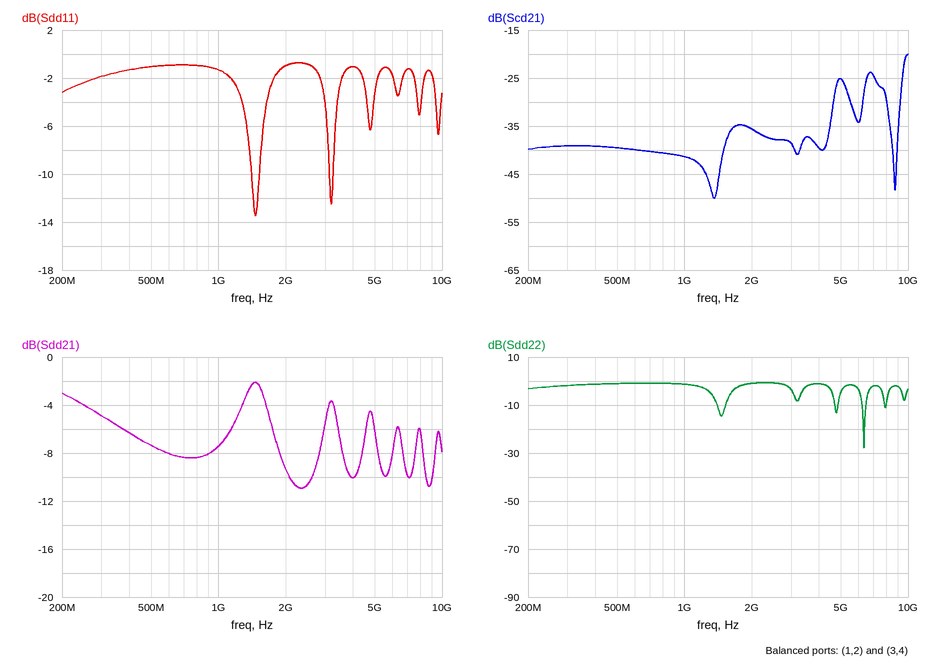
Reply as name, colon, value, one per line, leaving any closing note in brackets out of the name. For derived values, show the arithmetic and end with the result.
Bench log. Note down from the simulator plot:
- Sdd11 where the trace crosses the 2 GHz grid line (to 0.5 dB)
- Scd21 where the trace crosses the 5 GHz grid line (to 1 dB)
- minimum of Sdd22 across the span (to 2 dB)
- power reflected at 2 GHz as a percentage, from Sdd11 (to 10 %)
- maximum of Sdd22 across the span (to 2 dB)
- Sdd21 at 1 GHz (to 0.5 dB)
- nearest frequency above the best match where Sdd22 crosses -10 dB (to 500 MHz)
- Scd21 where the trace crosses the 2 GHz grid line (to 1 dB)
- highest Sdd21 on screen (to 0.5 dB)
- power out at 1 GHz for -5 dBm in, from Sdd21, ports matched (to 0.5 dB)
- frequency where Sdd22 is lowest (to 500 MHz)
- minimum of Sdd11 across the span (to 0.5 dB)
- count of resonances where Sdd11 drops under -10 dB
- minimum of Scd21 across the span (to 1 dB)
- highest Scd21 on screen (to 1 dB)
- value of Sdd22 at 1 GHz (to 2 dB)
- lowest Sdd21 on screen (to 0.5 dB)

Sdd11 where the trace crosses the 2 GHz grid line: -1.0 dB
Scd21 where the trace crosses the 5 GHz grid line: -25 dB
minimum of Sdd22 across the span: -28 dB
power reflected at 2 GHz as a percentage, from Sdd11: 10^(-1/10) ≈ 79.4 %, so 80 % to the nearest 10 %
maximum of Sdd22 across the span: 0 dB
Sdd21 at 1 GHz: -7.5 dB
nearest frequency above the best match where Sdd22 crosses -10 dB: 6.5 GHz
Scd21 where the trace crosses the 2 GHz grid line: -36 dB
highest Sdd21 on screen: -2.0 dB
power out at 1 GHz for -5 dBm in, from Sdd21, ports matched: -5 dBm + (-7.5 dB) = -12.5 dBm
frequency where Sdd22 is lowest: 6.5 GHz
minimum of Sdd11 across the span: -13.5 dB
count of resonances where Sdd11 drops under -10 dB: 2
minimum of Scd21 across the span: -50 dB
highest Scd21 on screen: -20 dB
value of Sdd22 at 1 GHz: -2 dB
lowest Sdd21 on screen: -11.0 dB
